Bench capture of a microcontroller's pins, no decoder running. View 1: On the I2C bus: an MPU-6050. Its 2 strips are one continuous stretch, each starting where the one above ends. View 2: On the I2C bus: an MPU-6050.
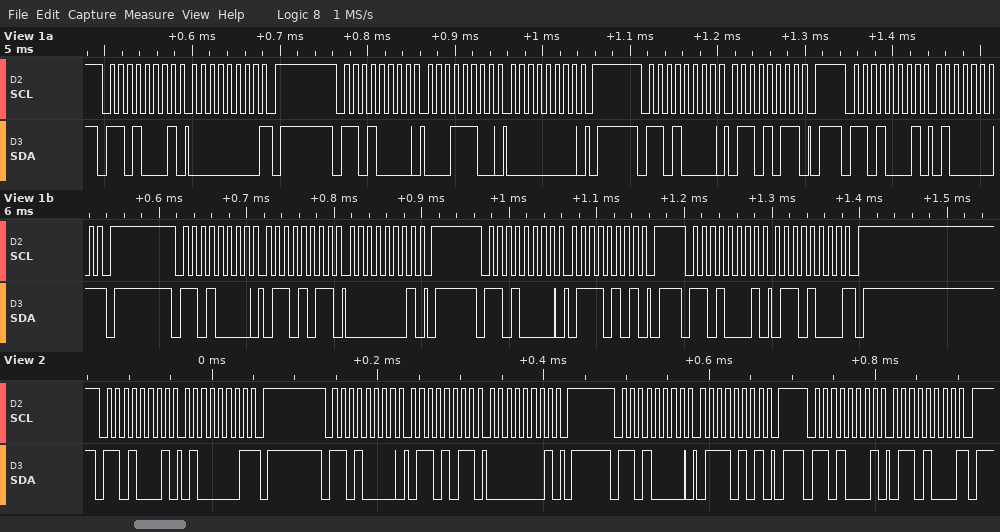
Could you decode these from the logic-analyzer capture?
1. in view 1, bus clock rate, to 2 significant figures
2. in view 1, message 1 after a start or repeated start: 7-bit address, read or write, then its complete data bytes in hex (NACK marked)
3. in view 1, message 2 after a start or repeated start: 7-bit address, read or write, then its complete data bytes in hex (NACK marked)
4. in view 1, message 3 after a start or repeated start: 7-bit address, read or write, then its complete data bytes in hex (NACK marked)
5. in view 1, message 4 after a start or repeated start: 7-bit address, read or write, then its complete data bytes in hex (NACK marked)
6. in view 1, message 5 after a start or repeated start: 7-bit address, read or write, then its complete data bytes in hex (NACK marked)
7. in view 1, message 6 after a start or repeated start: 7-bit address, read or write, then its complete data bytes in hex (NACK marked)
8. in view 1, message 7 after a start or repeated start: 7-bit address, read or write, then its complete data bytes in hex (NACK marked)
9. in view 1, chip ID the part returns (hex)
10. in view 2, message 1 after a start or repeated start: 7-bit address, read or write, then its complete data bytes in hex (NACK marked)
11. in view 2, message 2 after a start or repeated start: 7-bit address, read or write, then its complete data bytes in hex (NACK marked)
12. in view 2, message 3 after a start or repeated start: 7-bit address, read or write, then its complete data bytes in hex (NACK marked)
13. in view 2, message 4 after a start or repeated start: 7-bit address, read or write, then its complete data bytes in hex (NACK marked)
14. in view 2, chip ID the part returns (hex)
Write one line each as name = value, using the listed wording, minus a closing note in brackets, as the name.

in view 1, bus clock rate, to 2 significant figures = 100 kHz
in view 1, message 1 after a start or repeated start: 7-bit address, read or write, then its complete data bytes in hex = 0x68 read: 00 NACK
in view 1, message 2 after a start or repeated start: 7-bit address, read or write, then its complete data bytes in hex = 0x68 write: 1C 00
in view 1, message 3 after a start or repeated start: 7-bit address, read or write, then its complete data bytes in hex = 0x68 write: 6B
in view 1, message 4 after a start or repeated start: 7-bit address, read or write, then its complete data bytes in hex = 0x68 read: 41 NACK
in view 1, message 5 after a start or repeated start: 7-bit address, read or write, then its complete data bytes in hex = 0x68 write: 6B 01
in view 1, message 6 after a start or repeated start: 7-bit address, read or write, then its complete data bytes in hex = 0x68 write: 75
in view 1, message 7 after a start or repeated start: 7-bit address, read or write, then its complete data bytes in hex = 0x68 read: 68 NACK
in view 1, chip ID the part returns = 0x68
in view 2, message 1 after a start or repeated start: 7-bit address, read or write, then its complete data bytes in hex = 0x68 read: 41 NACK
in view 2, message 2 after a start or repeated start: 7-bit address, read or write, then its complete data bytes in hex = 0x68 write: 6B 01
in view 2, message 3 after a start or repeated start: 7-bit address, read or write, then its complete data bytes in hex = 0x68 write: 75
in view 2, message 4 after a start or repeated start: 7-bit address, read or write, then its complete data bytes in hex = 0x68 read: 68 NACK
in view 2, chip ID the part returns = 0x68
